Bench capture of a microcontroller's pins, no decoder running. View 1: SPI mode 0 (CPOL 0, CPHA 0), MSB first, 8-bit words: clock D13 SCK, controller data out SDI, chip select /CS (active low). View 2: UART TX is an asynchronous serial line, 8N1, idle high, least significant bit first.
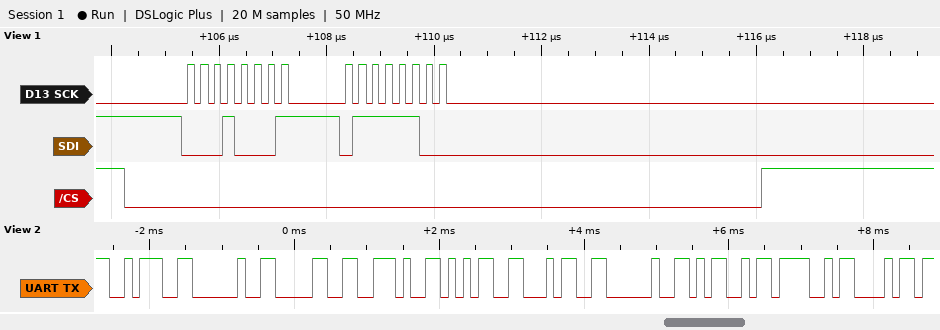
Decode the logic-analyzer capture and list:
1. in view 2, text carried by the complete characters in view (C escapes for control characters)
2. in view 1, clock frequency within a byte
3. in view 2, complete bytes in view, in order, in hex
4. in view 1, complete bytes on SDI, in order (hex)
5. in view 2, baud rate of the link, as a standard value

": 0.54 MOh"
4 MHz
0x3A 0x20 0x30 0x2E 0x35 0x34 0x20 0x4D 0x4F 0x68
0x11 0x7C
9600 baud
